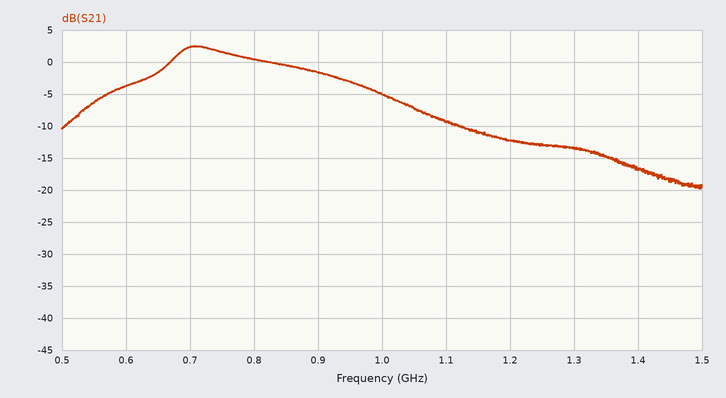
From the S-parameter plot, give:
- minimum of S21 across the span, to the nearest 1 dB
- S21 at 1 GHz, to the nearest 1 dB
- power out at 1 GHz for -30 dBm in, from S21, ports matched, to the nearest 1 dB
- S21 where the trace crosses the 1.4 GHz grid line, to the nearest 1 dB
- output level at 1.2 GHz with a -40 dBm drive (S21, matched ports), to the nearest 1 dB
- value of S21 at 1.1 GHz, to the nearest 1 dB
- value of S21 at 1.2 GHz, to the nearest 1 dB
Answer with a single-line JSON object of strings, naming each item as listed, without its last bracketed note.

{"minimum of S21 across the span, to the nearest 1 dB": "-20 dB", "S21 at 1 GHz, to the nearest 1 dB": "-5 dB", "power out at 1 GHz for -30 dBm in, from S21, ports matched, to the nearest 1 dB": "-35 dBm", "S21 where the trace crosses the 1.4 GHz grid line, to the nearest 1 dB": "-17 dB", "output level at 1.2 GHz with a -40 dBm drive (S21, matched ports), to the nearest 1 dB": "-52 dBm", "value of S21 at 1.1 GHz, to the nearest 1 dB": "-9 dB", "value of S21 at 1.2 GHz, to the nearest 1 dB": "-12 dB"}
